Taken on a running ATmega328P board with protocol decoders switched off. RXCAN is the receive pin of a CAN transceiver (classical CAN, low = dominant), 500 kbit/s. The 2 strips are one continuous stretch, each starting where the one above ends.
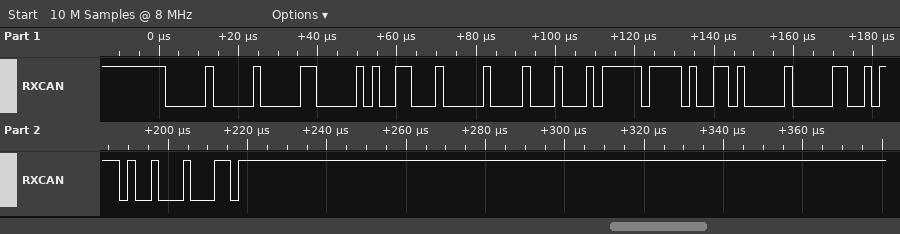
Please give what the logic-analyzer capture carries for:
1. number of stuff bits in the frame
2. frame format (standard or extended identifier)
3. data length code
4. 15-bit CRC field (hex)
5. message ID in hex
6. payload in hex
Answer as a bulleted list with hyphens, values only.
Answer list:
- 8
- standard
- 8
- 0x6911
- 0x000
- 13 10 04 45 FF 4D 00 25
